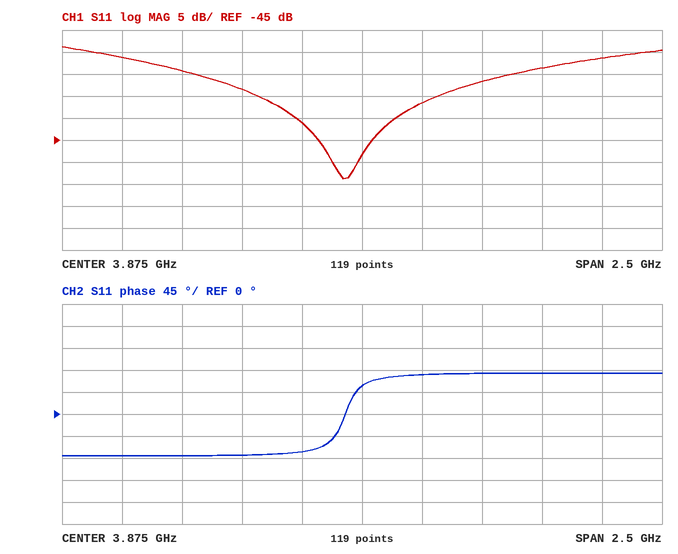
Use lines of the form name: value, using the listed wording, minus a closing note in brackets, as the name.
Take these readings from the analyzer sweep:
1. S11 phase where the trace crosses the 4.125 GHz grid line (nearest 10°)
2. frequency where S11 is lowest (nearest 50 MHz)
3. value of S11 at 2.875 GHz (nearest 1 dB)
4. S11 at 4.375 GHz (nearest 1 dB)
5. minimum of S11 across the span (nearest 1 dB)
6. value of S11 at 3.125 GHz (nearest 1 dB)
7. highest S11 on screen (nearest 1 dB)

S11 phase where the trace crosses the 4.125 GHz grid line: 80°
frequency where S11 is lowest: 3.80 GHz
value of S11 at 2.875 GHz: -26 dB
S11 at 4.375 GHz: -32 dB
minimum of S11 across the span: -54 dB
value of S11 at 3.125 GHz: -29 dB
highest S11 on screen: -24 dB
